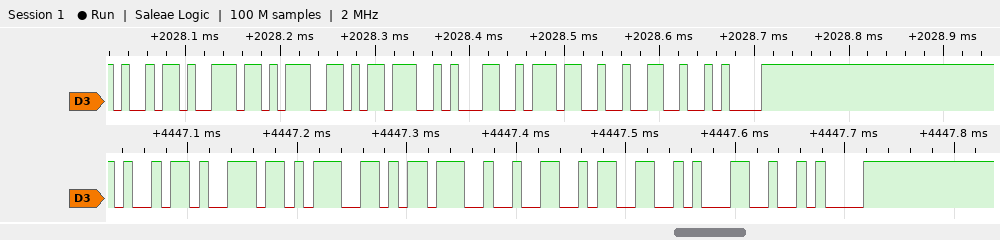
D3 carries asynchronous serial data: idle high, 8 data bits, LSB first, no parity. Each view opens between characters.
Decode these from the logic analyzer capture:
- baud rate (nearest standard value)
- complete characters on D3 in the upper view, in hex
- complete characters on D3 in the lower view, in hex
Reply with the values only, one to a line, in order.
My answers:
115200 baud
69, 6E, 67, 3B, 31, 37, 32, 0A
69, 6E, 67, 3B, 32, 33, 31, 0A
